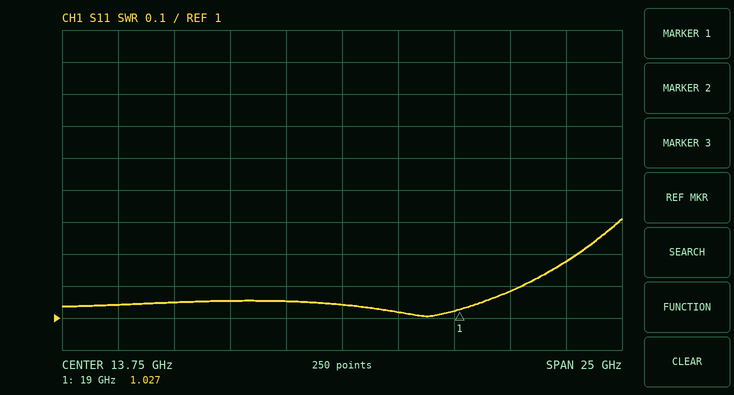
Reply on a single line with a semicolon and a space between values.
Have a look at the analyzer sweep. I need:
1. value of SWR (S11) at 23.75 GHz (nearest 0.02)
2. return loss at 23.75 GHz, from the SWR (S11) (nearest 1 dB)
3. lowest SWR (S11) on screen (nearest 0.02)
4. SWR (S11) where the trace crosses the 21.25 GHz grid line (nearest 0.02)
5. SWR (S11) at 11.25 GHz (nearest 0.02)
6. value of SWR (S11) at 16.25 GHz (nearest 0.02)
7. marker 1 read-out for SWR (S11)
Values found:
1.18; 22 dB; 1.00; 1.08; 1.06; 1.02; 1.027
